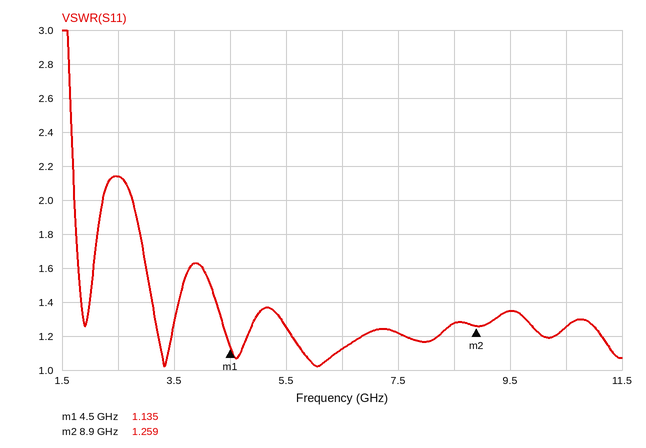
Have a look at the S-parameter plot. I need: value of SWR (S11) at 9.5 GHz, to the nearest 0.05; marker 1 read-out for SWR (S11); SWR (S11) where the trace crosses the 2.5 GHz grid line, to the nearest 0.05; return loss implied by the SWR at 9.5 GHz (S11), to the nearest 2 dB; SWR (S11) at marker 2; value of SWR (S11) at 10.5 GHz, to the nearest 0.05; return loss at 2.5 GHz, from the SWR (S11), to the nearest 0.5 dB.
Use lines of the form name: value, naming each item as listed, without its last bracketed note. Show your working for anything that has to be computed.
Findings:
value of SWR (S11) at 9.5 GHz, to the nearest 0.05: 1.35
marker 1 read-out for SWR: 1.135
SWR (S11) where the trace crosses the 2.5 GHz grid line, to the nearest 0.05: 2.15
return loss implied by the SWR at 9.5 GHz (S11), to the nearest 2 dB: −20 log10((1.35 − 1)/(1.35 + 1)) ≈ 16 dB
SWR (S11) at marker 2: 1.259
value of SWR (S11) at 10.5 GHz, to the nearest 0.05: 1.25
return loss at 2.5 GHz, from the SWR (S11), to the nearest 0.5 dB: −20 log10((2.15 − 1)/(2.15 + 1)) ≈ 8.75 dB, so 9.0 dB to the nearest 0.5 dB
